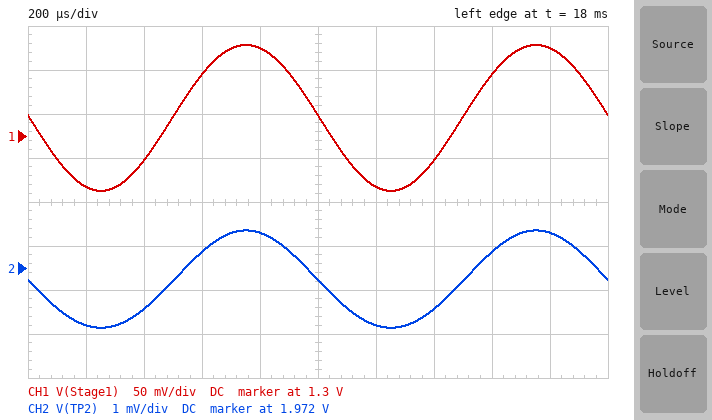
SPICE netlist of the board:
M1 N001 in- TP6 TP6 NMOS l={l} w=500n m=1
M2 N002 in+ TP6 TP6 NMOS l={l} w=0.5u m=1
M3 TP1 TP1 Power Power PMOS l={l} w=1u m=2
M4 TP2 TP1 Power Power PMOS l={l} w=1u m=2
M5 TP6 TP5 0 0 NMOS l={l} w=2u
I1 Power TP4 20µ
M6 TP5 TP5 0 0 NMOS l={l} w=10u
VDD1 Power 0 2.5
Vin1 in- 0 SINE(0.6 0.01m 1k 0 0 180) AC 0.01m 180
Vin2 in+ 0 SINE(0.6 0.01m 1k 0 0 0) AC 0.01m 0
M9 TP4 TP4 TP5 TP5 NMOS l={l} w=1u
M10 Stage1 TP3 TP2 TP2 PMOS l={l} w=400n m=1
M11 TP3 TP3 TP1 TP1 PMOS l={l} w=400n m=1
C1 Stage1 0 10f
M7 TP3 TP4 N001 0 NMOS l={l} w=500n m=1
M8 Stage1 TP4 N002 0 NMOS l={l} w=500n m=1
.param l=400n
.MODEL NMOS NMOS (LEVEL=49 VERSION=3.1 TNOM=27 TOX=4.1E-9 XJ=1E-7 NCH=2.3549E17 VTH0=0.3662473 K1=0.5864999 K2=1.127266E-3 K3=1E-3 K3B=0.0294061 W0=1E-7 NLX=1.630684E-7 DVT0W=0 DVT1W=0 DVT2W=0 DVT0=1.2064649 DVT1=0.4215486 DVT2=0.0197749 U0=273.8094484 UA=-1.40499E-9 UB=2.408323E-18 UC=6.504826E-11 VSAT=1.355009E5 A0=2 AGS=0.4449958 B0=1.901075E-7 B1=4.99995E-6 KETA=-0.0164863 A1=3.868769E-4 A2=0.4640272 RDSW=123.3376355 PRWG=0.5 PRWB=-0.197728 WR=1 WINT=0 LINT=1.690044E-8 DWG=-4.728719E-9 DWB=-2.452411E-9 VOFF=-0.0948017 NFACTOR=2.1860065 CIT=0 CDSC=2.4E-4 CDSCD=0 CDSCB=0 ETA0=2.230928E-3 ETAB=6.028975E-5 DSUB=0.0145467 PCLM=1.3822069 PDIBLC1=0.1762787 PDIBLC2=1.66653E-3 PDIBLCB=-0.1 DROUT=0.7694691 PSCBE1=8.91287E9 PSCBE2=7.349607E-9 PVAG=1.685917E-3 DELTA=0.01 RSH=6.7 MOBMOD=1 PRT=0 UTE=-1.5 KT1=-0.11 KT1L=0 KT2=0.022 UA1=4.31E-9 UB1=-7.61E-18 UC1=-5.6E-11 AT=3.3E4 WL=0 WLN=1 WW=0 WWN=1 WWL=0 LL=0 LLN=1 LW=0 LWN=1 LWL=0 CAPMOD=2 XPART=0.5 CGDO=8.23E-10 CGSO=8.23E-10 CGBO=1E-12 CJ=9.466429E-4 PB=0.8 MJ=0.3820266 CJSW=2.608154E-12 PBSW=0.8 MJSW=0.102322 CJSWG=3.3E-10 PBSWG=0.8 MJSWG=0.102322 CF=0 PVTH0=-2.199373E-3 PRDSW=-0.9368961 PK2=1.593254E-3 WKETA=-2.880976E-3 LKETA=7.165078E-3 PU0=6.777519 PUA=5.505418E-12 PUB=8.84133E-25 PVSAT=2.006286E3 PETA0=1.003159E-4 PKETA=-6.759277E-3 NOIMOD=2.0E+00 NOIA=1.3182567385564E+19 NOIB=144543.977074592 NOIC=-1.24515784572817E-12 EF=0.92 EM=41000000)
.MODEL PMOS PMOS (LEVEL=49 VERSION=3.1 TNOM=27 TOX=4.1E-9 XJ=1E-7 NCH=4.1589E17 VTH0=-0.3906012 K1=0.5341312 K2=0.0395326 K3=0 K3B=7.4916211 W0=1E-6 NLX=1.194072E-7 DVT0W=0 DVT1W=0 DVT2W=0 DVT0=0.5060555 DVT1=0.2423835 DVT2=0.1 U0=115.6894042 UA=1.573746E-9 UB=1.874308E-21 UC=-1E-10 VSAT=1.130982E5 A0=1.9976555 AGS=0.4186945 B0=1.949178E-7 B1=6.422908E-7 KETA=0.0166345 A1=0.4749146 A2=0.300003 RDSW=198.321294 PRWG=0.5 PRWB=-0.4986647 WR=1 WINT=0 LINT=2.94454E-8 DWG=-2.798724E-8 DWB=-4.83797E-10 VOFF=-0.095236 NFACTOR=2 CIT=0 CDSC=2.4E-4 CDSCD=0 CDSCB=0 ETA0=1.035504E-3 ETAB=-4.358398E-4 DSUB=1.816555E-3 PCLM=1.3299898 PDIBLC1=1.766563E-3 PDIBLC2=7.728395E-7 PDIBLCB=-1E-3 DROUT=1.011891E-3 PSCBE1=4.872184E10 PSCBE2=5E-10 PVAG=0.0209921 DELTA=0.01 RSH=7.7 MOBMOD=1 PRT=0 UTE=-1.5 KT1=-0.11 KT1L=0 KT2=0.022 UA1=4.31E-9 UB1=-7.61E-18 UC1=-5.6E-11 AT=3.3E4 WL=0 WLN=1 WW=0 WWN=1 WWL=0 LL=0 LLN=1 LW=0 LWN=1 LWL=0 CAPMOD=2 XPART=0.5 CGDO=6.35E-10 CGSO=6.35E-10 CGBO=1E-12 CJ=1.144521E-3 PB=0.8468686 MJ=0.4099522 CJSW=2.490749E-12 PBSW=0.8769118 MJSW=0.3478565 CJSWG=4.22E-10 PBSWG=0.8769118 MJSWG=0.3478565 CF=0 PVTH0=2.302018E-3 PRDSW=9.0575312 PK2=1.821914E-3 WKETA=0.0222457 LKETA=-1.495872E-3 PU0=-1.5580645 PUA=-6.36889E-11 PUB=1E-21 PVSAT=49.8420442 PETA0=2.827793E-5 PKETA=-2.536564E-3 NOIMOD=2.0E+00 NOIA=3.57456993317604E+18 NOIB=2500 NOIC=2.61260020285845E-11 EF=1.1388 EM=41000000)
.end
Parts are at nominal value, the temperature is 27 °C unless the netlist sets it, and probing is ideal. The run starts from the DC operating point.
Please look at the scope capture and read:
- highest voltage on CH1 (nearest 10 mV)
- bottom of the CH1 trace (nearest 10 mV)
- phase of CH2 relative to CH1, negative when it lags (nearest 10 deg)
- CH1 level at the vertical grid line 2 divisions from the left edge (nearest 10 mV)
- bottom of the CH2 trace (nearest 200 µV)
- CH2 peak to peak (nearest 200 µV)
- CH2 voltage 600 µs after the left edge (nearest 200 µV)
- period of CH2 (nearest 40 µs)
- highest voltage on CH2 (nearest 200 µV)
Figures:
1.40 V
1.24 V
0 deg
1.27 V
1.9706 V
2.2 mV
1.9724 V
1.00 ms
1.9728 V
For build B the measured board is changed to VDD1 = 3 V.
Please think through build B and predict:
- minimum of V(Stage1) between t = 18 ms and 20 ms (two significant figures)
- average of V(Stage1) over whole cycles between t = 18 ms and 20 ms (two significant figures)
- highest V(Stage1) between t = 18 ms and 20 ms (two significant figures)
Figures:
1.7 V
1.8 V
1.9 V
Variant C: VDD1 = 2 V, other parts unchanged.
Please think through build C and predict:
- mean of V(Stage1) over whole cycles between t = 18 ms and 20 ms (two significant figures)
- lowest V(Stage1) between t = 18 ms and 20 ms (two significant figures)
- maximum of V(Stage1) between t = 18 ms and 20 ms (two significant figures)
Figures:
820 mV
770 mV
890 mV
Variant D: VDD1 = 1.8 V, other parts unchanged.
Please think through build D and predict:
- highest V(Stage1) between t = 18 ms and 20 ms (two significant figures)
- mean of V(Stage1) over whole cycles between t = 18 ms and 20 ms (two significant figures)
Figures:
630 mV
620 mV
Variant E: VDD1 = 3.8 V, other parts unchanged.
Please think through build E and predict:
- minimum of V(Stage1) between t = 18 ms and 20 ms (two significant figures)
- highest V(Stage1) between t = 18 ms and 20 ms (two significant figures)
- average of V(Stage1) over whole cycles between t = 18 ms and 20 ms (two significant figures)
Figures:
2.5 V
2.7 V
2.6 V
